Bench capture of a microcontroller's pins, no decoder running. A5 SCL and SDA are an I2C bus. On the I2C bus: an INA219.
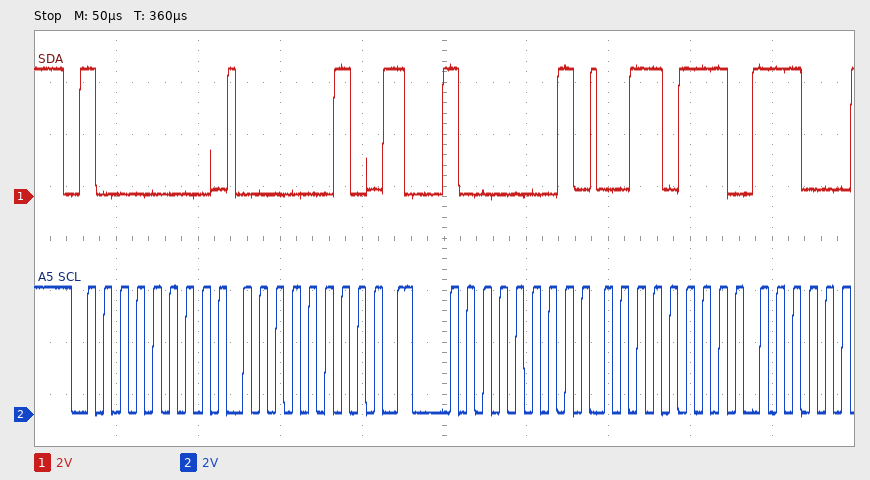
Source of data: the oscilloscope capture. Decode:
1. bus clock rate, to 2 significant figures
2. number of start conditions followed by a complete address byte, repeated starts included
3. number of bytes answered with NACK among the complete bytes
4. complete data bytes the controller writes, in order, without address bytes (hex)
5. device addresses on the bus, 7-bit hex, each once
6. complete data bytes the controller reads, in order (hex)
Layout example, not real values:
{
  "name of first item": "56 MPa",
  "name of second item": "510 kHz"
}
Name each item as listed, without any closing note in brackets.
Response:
{
  "bus clock rate, to 2 significant figures": "100 kHz",
  "number of start conditions followed by a complete address byte, repeated starts included": "2",
  "number of bytes answered with NACK among the complete bytes": "0",
  "complete data bytes the controller writes, in order, without address bytes": "02",
  "device addresses on the bus, 7-bit hex, each once": "0x40",
  "complete data bytes the controller reads, in order": "37"
}
